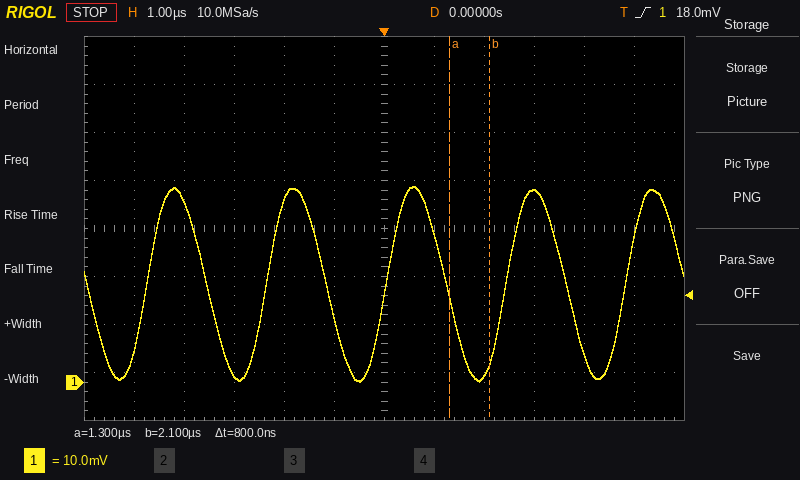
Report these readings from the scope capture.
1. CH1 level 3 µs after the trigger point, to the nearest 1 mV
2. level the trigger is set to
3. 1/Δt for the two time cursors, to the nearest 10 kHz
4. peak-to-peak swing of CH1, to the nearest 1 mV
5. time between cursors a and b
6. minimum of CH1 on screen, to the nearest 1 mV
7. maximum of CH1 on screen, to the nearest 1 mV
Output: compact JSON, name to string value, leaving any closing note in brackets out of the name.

{"CH1 level 3 µs after the trigger point, to the nearest 1 mV": "40 mV", "level the trigger is set to": "18.0 mV", "1/Δt for the two time cursors, to the nearest 10 kHz": "1.25 MHz", "peak-to-peak swing of CH1, to the nearest 1 mV": "41 mV", "time between cursors a and b": "800 ns", "minimum of CH1 on screen, to the nearest 1 mV": "0 mV", "maximum of CH1 on screen, to the nearest 1 mV": "41 mV"}
